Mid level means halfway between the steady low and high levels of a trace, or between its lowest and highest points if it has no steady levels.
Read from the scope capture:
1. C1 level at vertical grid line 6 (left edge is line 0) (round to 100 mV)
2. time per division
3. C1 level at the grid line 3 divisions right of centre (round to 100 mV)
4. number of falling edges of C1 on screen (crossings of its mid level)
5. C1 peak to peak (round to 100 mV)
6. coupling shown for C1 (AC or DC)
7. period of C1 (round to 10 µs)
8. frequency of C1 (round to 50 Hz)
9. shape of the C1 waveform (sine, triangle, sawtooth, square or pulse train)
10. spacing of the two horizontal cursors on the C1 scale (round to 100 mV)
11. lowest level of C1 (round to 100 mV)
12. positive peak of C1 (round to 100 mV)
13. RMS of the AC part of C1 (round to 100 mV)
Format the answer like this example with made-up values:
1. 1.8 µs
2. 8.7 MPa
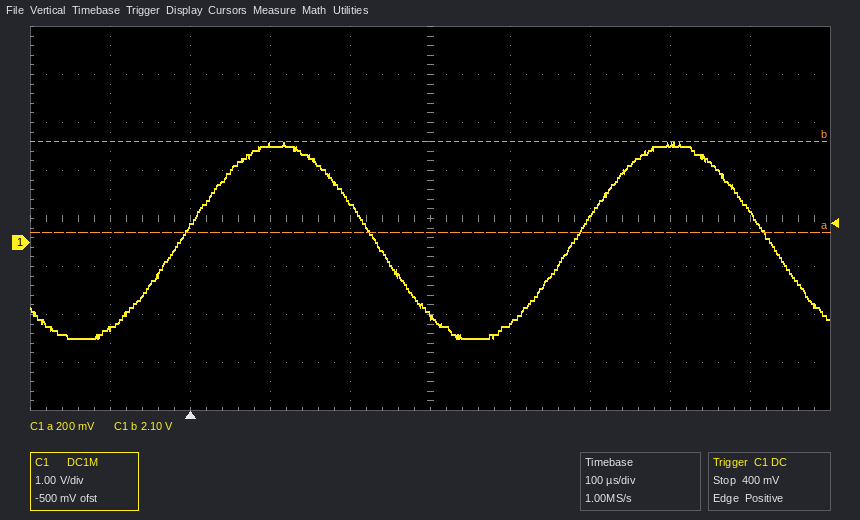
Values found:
1. -1.7 V
2. 100 µs
3. 2.0 V
4. 2
5. 4.1 V
6. DC
7. 490 µs
8. 2.05 kHz
9. sine
10. 1.9 V
11. -2.0 V
12. 2.1 V
13. 1.4 V
